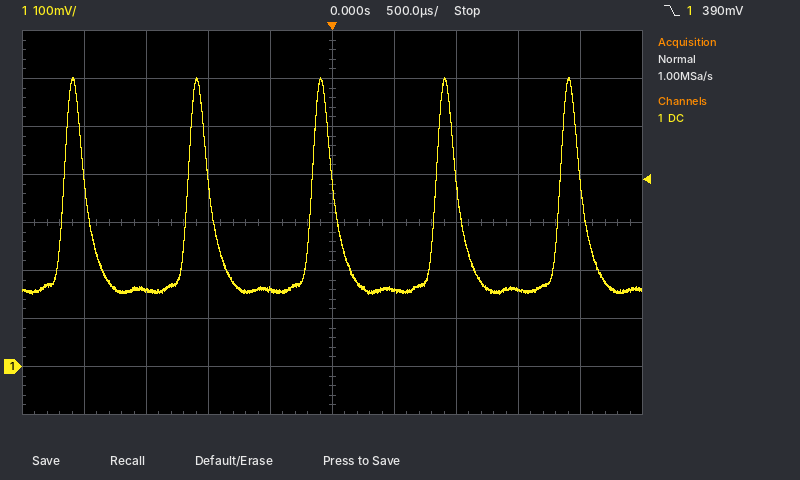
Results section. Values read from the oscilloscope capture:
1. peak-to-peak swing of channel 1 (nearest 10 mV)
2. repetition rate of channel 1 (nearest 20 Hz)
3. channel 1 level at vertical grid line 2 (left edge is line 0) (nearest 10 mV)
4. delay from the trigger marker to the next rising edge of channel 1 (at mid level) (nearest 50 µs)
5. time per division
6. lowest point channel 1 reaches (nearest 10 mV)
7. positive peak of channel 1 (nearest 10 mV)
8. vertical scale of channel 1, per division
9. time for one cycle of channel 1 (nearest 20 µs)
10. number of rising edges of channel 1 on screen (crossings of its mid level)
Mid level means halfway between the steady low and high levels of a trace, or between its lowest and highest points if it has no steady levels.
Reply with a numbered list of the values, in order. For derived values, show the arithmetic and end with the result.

1. 600 mV − (150 mV) = 450 mV
2. 1 / 1.00 ms ≈ 1.00 kHz
3. 160 mV
4. 850 µs
5. 500 µs
6. 150 mV
7. 600 mV
8. 100 mV
9. 1.00 ms
10. 5
